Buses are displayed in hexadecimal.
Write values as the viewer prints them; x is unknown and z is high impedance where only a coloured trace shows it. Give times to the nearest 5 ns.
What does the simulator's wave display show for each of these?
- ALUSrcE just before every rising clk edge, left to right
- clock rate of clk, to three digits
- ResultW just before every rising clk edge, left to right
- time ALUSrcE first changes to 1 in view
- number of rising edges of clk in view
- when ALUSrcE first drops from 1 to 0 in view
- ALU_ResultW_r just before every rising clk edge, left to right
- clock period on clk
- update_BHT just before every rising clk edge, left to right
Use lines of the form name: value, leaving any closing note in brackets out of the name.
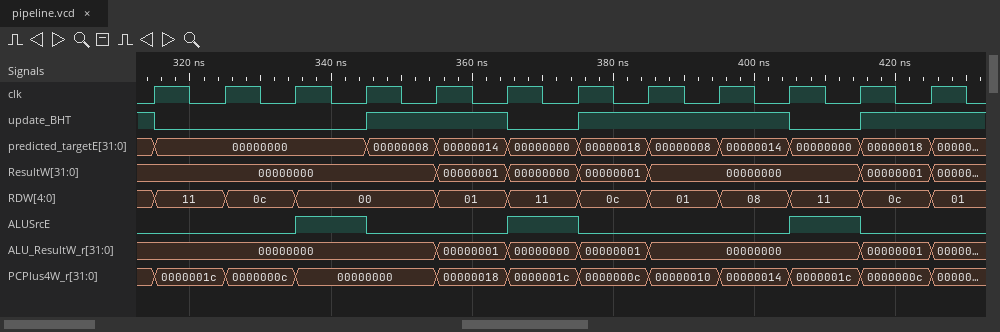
ALUSrcE just before every rising clk edge, left to right: 0 0 0 1 0 0 1 0 0 0 1 0
clock rate of clk, to three digits: 100 MHz
ResultW just before every rising clk edge, left to right: 00000000, 00000000, 00000000, 00000000, 00000000, 00000001, 00000000, 00000001, 00000000, 00000000, 00000000, 00000001
time ALUSrcE first changes to 1 in view: 335 ns
number of rising edges of clk in view: 12
when ALUSrcE first drops from 1 to 0 in view: 345 ns
ALU_ResultW_r just before every rising clk edge, left to right: 00000000, 00000000, 00000000, 00000000, 00000000, 00000001, 00000000, 00000001, 00000000, 00000000, 00000000, 00000001
clock period on clk: 10 ns
update_BHT just before every rising clk edge, left to right: 1 0 0 0 1 1 0 1 1 1 0 1
